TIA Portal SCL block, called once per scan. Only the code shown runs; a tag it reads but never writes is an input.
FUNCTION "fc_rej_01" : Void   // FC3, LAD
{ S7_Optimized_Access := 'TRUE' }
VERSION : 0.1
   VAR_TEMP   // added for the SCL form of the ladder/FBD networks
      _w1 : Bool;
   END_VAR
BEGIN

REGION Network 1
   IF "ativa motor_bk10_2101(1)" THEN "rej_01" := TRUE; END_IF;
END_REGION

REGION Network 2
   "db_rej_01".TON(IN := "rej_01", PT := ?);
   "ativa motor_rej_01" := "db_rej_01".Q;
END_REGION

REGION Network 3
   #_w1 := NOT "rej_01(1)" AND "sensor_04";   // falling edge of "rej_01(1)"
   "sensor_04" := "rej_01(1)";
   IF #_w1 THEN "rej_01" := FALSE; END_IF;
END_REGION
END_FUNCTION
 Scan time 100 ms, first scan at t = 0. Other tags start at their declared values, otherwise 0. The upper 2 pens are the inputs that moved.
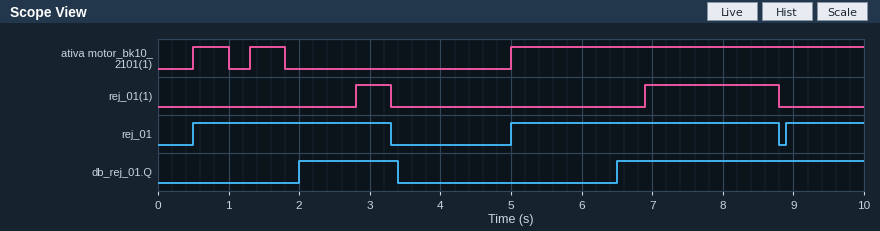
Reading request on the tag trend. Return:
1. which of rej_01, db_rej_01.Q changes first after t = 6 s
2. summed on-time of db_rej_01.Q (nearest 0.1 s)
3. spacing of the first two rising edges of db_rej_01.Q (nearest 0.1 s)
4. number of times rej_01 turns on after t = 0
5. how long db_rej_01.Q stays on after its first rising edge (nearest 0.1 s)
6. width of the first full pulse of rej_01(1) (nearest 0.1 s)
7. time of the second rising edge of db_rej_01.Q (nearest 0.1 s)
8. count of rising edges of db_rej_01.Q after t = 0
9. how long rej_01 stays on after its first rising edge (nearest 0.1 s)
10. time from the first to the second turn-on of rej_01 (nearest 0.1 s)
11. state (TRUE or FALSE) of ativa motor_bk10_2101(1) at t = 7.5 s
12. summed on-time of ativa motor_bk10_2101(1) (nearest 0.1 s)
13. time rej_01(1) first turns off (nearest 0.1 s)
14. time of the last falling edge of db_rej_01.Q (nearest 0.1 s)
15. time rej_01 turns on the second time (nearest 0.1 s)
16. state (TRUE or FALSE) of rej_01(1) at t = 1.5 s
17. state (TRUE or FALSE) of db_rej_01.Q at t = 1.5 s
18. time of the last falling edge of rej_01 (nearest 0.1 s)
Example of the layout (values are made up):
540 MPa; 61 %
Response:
db_rej_01.Q; 4.9 s; 4.5 s; 3; 1.4 s; 0.5 s; 6.5 s; 2; 2.8 s; 4.5 s; TRUE; 6.0 s; 3.3 s; 3.4 s; 5.0 s; FALSE; FALSE; 8.8 s
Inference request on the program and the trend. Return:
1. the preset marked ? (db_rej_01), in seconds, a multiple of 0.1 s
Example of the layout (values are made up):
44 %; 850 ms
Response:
1.5 s
